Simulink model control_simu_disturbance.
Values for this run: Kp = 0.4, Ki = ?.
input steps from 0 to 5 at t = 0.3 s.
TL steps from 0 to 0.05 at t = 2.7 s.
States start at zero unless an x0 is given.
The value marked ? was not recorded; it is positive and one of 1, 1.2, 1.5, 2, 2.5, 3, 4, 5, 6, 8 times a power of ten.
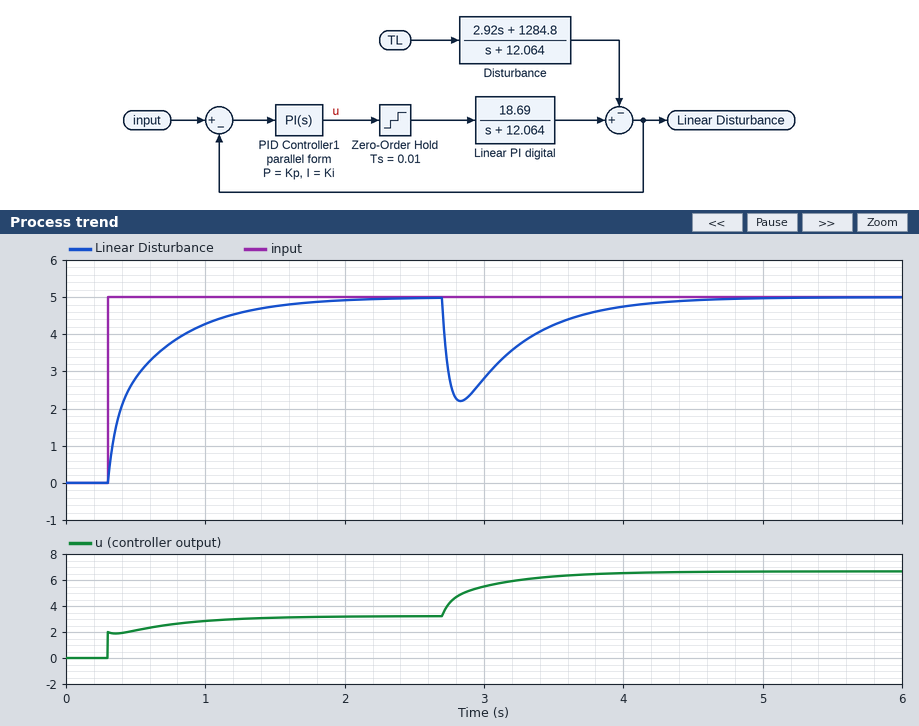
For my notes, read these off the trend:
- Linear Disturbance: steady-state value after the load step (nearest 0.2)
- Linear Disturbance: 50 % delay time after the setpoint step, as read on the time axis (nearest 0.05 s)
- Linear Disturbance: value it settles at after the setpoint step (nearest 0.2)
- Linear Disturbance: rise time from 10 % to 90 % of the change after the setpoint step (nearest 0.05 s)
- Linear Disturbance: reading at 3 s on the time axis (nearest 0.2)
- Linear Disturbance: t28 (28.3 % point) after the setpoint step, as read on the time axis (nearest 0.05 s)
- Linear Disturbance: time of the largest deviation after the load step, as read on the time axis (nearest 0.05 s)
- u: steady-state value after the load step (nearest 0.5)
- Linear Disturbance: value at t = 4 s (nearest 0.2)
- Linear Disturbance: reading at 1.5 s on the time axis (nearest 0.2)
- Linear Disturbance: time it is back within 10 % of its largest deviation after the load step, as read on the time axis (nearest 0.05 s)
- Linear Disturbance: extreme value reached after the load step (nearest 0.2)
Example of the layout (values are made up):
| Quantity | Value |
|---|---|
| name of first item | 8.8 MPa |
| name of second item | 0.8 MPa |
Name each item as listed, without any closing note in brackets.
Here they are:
| Quantity | Value |
|---|---|
| Linear Disturbance: steady-state value after the load step | 5.0 |
| Linear Disturbance: 50 % delay time after the setpoint step, as read on the time axis | 0.45 s |
| Linear Disturbance: value it settles at after the setpoint step | 5.0 |
| Linear Disturbance: rise time from 10 % to 90 % of the change after the setpoint step | 0.85 s |
| Linear Disturbance: reading at 3 s on the time axis | 2.8 |
| Linear Disturbance: t28 (28.3 % point) after the setpoint step, as read on the time axis | 0.35 s |
| Linear Disturbance: time of the largest deviation after the load step, as read on the time axis | 2.85 s |
| u: steady-state value after the load step | 6.5 |
| Linear Disturbance: value at t = 4 s | 4.8 |
| Linear Disturbance: reading at 1.5 s on the time axis | 4.8 |
| Linear Disturbance: time it is back within 10 % of its largest deviation after the load step, as read on the time axis | 3.95 s |
| Linear Disturbance: extreme value reached after the load step | 2.2 |
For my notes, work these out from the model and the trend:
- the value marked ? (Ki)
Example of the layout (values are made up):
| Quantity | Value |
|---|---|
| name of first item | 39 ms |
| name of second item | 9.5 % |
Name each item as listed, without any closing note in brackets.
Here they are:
| Quantity | Value |
|---|---|
| the value marked ? | 2 |
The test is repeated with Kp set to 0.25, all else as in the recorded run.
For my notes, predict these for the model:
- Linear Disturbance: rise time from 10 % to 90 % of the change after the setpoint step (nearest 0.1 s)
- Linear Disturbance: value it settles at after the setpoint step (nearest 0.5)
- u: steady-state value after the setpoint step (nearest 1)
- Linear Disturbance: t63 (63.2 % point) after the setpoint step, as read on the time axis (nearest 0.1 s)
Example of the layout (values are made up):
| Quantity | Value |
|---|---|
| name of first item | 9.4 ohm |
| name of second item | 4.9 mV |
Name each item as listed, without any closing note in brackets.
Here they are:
| Quantity | Value |
|---|---|
| Linear Disturbance: rise time from 10 % to 90 % of the change after the setpoint step | 0.8 s |
| Linear Disturbance: value it settles at after the setpoint step | 5.0 |
| u: steady-state value after the setpoint step | 3 |
| Linear Disturbance: t63 (63.2 % point) after the setpoint step, as read on the time axis | 0.6 s |
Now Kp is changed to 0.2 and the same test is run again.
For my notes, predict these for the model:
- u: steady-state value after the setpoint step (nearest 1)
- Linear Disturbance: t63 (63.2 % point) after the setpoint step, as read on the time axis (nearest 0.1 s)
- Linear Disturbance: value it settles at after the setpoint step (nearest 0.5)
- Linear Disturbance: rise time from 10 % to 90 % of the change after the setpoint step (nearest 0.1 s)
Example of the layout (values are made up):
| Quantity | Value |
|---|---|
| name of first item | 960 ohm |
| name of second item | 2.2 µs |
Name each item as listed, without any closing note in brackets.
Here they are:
| Quantity | Value |
|---|---|
| u: steady-state value after the setpoint step | 3 |
| Linear Disturbance: t63 (63.2 % point) after the setpoint step, as read on the time axis | 0.6 s |
| Linear Disturbance: value it settles at after the setpoint step | 5.0 |
| Linear Disturbance: rise time from 10 % to 90 % of the change after the setpoint step | 0.7 s |
